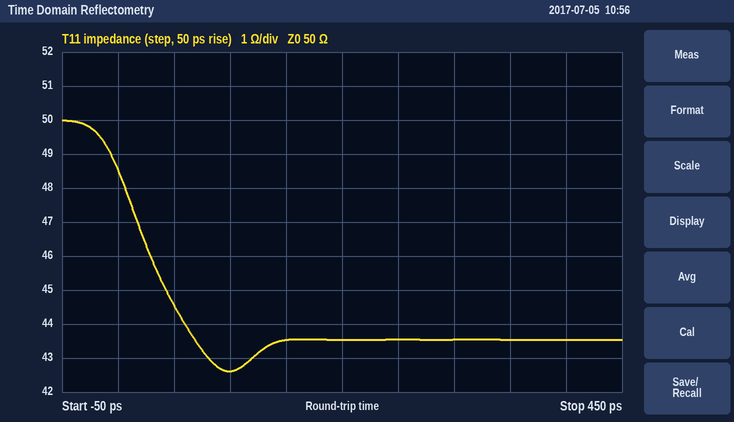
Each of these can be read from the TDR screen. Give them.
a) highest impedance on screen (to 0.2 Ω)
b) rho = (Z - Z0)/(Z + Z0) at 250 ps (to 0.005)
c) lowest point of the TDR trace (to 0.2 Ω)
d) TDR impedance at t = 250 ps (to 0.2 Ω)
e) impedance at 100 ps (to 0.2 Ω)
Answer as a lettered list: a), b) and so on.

a) 50.0 Ω
b) -0.070
c) 42.6 Ω
d) 43.6 Ω
e) 42.6 Ω
